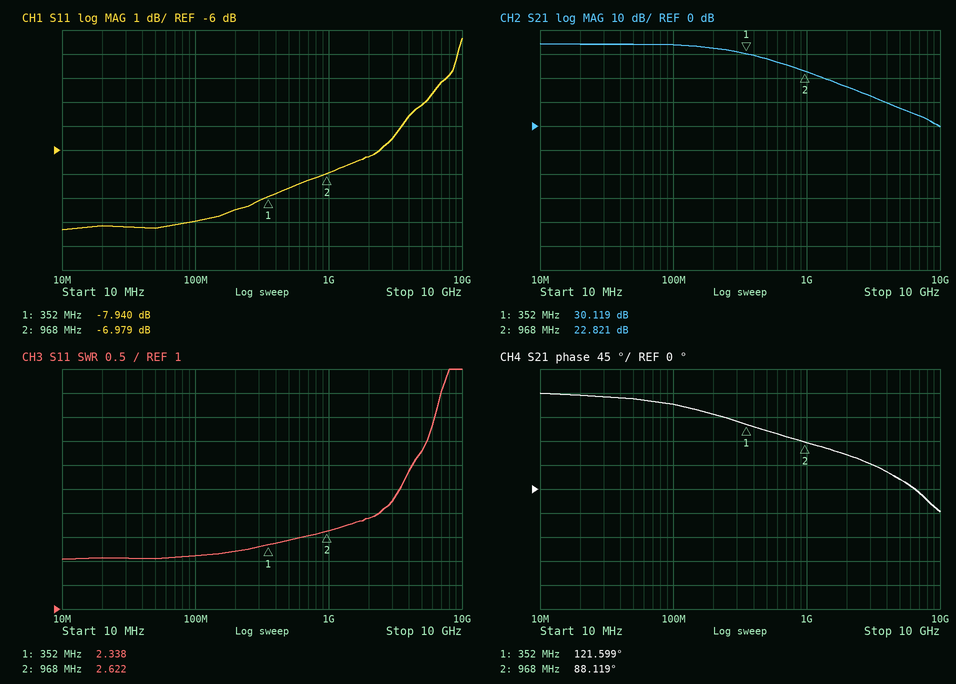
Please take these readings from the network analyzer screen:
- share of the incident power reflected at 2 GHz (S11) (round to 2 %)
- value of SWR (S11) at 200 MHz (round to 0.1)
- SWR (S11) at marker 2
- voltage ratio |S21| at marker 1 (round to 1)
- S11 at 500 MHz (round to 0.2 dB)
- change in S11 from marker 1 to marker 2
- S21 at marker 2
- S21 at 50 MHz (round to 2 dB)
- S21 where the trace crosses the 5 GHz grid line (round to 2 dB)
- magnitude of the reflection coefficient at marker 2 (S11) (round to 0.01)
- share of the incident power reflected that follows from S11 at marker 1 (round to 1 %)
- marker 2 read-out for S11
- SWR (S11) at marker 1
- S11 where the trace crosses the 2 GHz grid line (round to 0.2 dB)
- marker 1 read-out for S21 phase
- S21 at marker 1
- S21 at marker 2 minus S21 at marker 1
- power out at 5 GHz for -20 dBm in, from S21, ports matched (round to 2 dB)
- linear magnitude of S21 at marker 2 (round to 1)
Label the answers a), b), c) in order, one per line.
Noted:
a) 24 %
b) 2.2
c) 2.622
d) 32
e) -7.6 dB
f) 0.961 dB
g) 22.821 dB
h) 34 dB
i) 8 dB
j) 0.45
k) 16 %
l) -6.979 dB
m) 2.338
n) -6.2 dB
o) 121.599°
p) 30.119 dB
q) -7.298 dB
r) -12 dBm
s) 14
